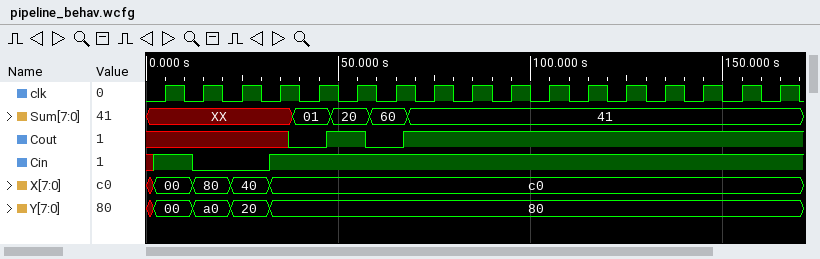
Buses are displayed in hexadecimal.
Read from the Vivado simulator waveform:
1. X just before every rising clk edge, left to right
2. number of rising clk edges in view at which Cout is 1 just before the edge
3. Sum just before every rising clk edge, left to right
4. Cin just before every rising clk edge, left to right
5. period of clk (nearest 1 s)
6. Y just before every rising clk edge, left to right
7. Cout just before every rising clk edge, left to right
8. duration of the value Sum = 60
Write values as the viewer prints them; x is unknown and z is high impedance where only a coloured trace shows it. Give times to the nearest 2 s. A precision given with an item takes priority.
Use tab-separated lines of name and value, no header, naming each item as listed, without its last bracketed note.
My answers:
X just before every rising clk edge, left to right	00, 80, 40, c0, c0, c0, c0, c0, c0, c0, c0, c0, c0, c0, c0, c0, c0
number of rising clk edges in view at which Cout is 1 just before the edge	11
Sum just before every rising clk edge, left to right	XX, XX, XX, XX, 01, 20, 60, 41, 41, 41, 41, 41, 41, 41, 41, 41, 41
Cin just before every rising clk edge, left to right	1 0 0 1 1 1 1 1 1 1 1 1 1 1 1 1 1
period of clk	10 s
Y just before every rising clk edge, left to right	00, a0, 20, 80, 80, 80, 80, 80, 80, 80, 80, 80, 80, 80, 80, 80, 80
Cout just before every rising clk edge, left to right	x x x x 0 1 0 1 1 1 1 1 1 1 1 1 1
duration of the value Sum = 60	10 s
